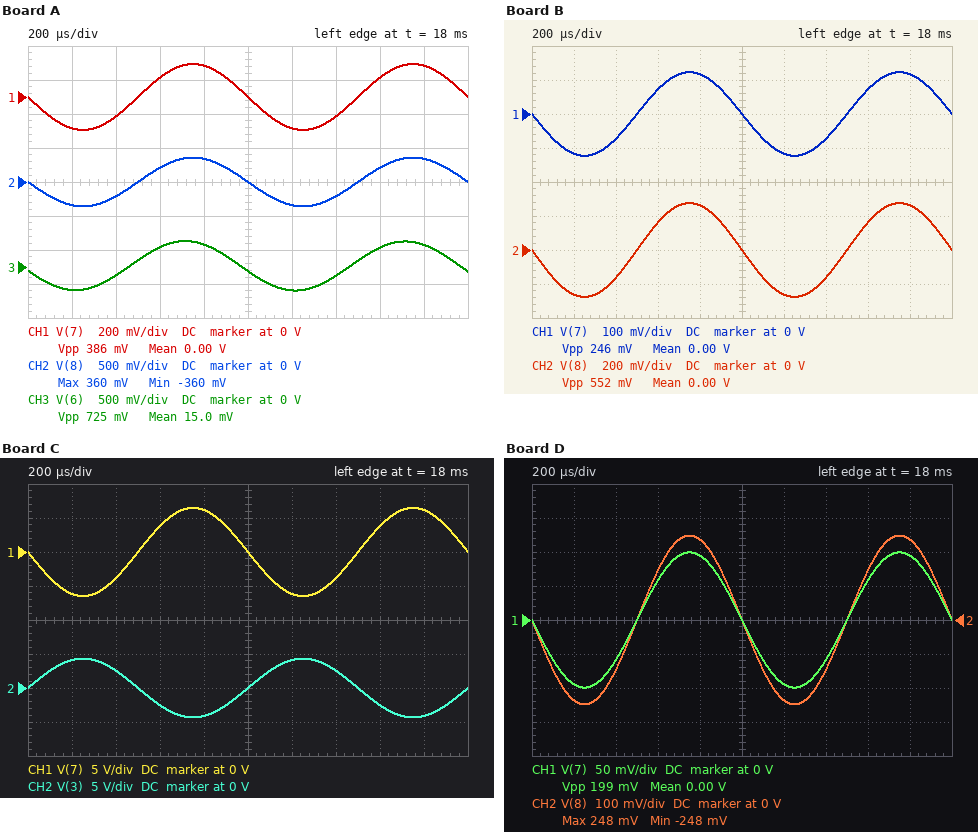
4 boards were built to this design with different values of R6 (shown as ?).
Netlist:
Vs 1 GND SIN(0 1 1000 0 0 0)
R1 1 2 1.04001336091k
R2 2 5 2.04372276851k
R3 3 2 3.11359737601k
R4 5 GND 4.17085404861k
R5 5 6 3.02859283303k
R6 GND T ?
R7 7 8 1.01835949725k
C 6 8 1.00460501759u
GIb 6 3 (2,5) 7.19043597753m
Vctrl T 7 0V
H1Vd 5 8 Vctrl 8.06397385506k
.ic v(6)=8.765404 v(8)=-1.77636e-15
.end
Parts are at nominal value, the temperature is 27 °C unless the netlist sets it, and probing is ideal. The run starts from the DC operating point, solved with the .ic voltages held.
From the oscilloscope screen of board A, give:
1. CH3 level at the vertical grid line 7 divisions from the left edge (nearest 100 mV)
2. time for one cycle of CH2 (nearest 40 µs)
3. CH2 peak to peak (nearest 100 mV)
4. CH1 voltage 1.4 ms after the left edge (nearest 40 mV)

-100 mV
1.00 ms
700 mV
-120 mV
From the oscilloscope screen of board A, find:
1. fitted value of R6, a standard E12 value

1.2 kΩ
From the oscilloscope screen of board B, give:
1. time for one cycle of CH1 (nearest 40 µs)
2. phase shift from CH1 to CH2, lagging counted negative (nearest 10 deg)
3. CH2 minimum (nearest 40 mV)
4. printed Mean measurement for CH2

1.00 ms
0 deg
-280 mV
0.00 V
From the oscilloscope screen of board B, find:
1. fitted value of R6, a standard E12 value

820 Ω
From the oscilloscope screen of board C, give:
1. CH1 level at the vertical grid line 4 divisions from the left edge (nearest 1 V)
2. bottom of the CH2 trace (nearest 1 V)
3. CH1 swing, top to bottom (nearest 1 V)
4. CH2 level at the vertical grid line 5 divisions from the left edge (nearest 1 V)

6 V
-4 V
13 V
0 V
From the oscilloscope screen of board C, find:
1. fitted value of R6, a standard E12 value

5.6 kΩ
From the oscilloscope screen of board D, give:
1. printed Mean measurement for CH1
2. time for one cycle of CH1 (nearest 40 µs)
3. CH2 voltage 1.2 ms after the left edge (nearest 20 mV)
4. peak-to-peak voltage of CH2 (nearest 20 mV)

0.00 V
1.00 ms
-240 mV
500 mV
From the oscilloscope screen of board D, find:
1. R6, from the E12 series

680 Ω
